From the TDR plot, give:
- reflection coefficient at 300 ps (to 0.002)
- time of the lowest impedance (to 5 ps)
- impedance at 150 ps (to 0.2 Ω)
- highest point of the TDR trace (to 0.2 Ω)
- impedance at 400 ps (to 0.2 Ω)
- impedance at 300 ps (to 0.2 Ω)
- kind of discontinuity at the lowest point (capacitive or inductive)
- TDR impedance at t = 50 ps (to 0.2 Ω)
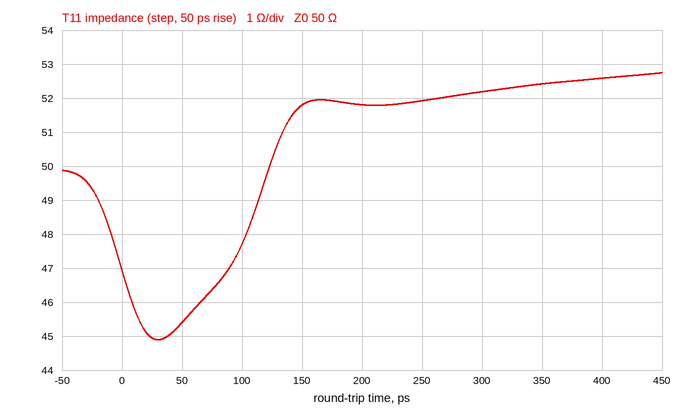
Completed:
+0.022
30 ps
51.8 Ω
52.8 Ω
52.6 Ω
52.2 Ω
capacitive
45.4 Ω
